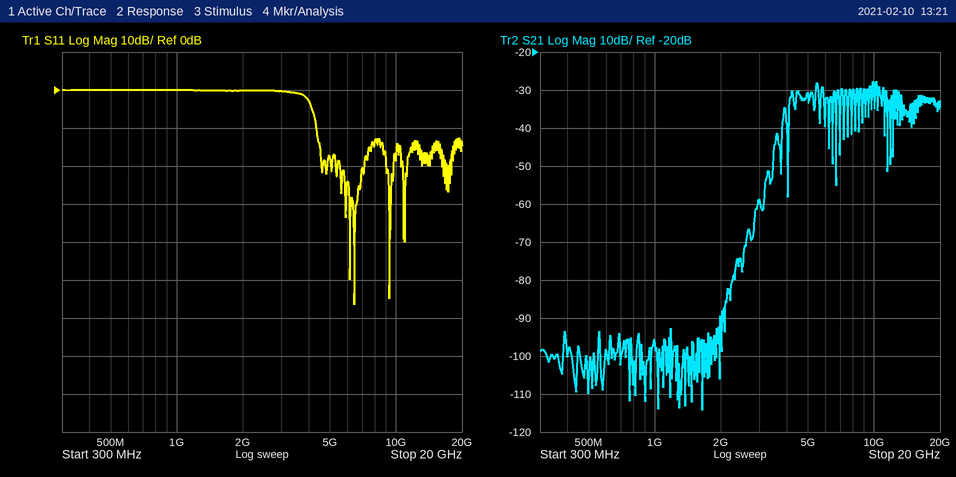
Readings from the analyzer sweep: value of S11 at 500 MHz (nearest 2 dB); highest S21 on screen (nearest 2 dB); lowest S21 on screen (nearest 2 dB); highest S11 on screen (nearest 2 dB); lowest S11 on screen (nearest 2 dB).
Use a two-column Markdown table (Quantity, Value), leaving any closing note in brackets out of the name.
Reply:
| Quantity | Value |
|---|---|
| value of S11 at 500 MHz | 0 dB |
| highest S21 on screen | -28 dB |
| lowest S21 on screen | -114 dB |
| highest S11 on screen | 0 dB |
| lowest S11 on screen | -56 dB |
